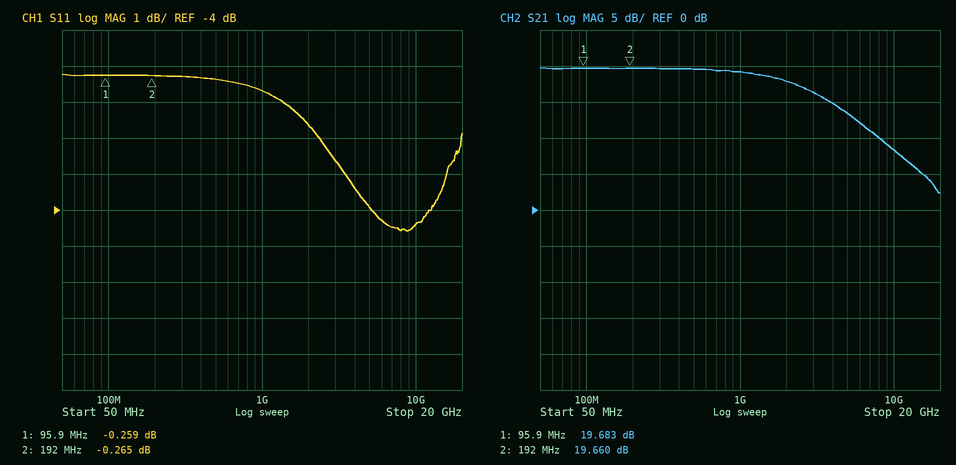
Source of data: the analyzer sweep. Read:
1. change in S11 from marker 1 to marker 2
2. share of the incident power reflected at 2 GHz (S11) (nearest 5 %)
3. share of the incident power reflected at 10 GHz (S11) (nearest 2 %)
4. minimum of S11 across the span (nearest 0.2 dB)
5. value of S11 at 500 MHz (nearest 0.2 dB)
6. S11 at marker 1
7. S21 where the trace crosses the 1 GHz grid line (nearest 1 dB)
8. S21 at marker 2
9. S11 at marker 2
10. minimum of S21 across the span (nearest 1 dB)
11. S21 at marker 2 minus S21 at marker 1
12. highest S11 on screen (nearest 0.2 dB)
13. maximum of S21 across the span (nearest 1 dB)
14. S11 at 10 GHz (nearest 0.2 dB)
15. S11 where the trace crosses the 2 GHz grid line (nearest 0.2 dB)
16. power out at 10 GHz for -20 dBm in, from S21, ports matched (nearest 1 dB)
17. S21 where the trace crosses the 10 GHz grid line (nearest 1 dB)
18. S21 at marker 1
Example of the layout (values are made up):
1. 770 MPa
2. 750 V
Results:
1. -0.006 dB
2. 70 %
3. 36 %
4. -4.6 dB
5. -0.4 dB
6. -0.259 dB
7. 19 dB
8. 19.660 dB
9. -0.265 dB
10. 2 dB
11. -0.023 dB
12. -0.2 dB
13. 20 dB
14. -4.4 dB
15. -1.6 dB
16. -12 dBm
17. 8 dB
18. 19.683 dB
